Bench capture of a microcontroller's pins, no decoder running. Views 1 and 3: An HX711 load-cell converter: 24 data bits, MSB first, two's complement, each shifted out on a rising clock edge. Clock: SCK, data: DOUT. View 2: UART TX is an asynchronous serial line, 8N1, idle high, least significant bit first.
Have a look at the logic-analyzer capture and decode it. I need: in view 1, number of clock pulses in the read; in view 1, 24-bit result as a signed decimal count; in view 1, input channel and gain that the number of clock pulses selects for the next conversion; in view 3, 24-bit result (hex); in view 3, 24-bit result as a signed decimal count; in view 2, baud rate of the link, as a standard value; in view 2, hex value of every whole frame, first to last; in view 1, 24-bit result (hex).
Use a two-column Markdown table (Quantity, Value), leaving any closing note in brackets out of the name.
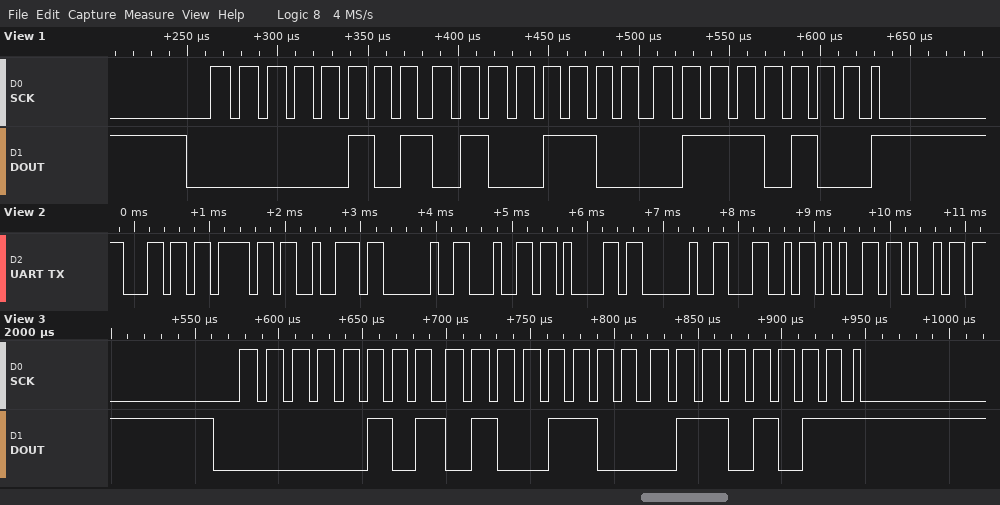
| Quantity | Value |
|---|---|
| in view 1, number of clock pulses in the read | 25 |
| in view 1, 24-bit result as a signed decimal count | 347252 |
| in view 1, input channel and gain that the number of clock pulses selects for the next conversion | channel A, gain 128 |
| in view 3, 24-bit result | 0x054C6B |
| in view 3, 24-bit result as a signed decimal count | 347243 |
| in view 2, baud rate of the link, as a standard value | 9600 baud |
| in view 2, hex value of every whole frame, first to last | 0x6C 0x6F 0x72 0x20 0x64 0x61 0x20 0x4C 0x65 0x69 |
| in view 1, 24-bit result | 0x054C74 |
